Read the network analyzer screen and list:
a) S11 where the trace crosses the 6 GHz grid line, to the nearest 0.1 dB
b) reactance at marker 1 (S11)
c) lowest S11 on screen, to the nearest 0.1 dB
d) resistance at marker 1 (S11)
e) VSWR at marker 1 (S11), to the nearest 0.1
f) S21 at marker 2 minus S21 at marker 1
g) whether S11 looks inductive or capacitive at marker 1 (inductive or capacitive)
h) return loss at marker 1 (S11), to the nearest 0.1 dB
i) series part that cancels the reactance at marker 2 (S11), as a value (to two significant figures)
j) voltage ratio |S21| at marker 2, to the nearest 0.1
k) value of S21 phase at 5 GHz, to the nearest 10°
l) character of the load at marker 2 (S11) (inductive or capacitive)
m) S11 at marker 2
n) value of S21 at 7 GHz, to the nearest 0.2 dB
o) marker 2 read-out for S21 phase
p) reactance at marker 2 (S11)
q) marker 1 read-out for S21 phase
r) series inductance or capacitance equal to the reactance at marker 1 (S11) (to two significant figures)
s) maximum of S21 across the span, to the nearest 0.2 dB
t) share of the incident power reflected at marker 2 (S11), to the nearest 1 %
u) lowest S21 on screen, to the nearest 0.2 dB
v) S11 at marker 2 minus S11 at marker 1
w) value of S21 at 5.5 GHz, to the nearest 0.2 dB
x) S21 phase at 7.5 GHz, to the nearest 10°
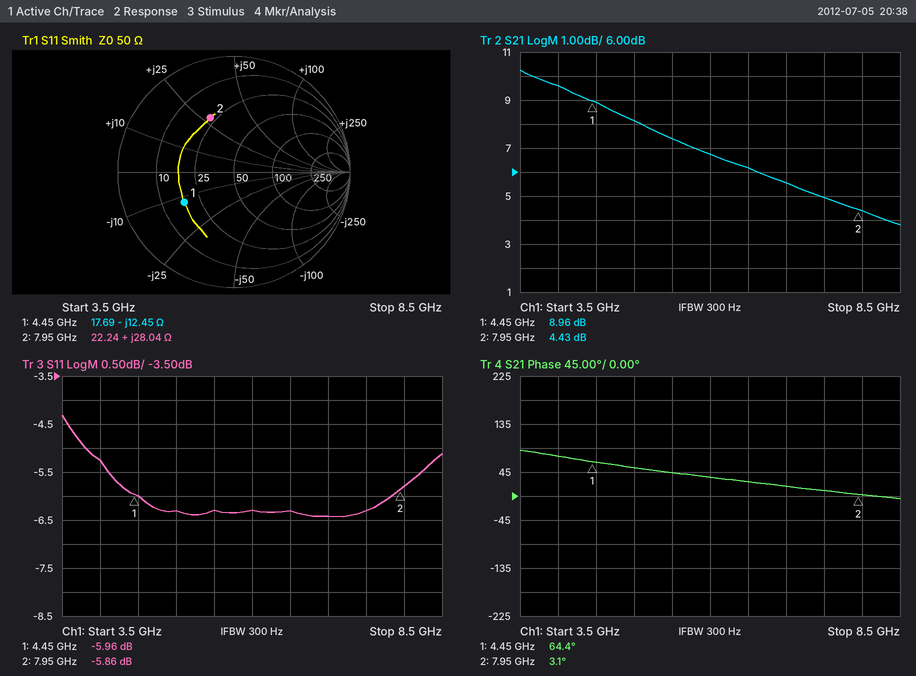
-6.3 dB
-12.45 Ω
-6.4 dB
17.69 Ω
3.0
-4.53 dB
capacitive
6.0 dB
710 fF
1.7
50°
inductive
-5.86 dB
5.6 dB
3.1°
+28.04 Ω
64.4°
2.9 pF
10.2 dB
26 %
3.8 dB
0.10 dB
7.4 dB
10°
